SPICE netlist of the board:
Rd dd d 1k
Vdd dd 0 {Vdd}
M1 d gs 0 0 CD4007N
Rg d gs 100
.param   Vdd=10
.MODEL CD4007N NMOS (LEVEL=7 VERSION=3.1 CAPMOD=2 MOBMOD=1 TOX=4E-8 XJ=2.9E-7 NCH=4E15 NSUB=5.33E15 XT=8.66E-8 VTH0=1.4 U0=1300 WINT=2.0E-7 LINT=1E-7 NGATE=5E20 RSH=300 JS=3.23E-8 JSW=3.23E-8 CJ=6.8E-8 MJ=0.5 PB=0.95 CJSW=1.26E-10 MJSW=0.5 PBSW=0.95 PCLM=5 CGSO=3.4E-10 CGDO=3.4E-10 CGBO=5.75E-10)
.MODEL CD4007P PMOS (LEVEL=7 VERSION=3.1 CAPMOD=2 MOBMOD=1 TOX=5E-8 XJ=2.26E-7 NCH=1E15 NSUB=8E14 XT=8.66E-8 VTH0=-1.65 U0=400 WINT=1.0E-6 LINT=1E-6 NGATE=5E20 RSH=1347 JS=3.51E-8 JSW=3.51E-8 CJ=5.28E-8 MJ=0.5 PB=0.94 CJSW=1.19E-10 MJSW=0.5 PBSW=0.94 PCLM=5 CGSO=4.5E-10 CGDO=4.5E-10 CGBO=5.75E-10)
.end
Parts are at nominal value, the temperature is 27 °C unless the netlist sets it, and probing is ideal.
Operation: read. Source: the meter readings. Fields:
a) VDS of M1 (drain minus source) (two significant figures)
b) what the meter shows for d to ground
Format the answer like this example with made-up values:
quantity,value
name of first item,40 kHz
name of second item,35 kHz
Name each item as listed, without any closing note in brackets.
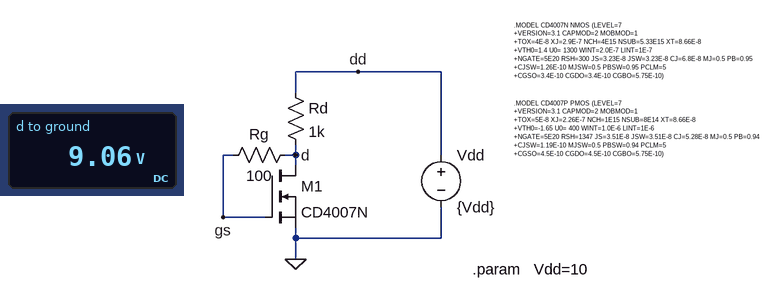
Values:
quantity,value
VDS of M1 (drain minus source),9.1 V
what the meter shows for d to ground,9.06 V
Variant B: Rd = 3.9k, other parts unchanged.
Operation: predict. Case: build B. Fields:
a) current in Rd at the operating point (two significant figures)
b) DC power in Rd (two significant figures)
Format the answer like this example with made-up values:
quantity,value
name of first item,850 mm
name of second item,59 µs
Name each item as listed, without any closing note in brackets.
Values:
quantity,value
current in Rd at the operating point,650 µA
DC power in Rd,1.7 mW
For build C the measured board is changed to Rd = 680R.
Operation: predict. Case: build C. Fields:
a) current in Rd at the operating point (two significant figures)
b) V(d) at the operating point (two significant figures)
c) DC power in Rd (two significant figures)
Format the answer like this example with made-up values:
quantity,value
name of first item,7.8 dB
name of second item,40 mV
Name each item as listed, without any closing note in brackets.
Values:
quantity,value
current in Rd at the operating point,990 µA
V(d) at the operating point,9.3 V
DC power in Rd,660 µW
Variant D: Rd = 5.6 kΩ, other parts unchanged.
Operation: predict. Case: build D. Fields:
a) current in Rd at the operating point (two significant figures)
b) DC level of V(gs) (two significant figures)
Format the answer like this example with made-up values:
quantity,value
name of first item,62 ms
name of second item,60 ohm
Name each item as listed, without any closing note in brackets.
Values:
quantity,value
current in Rd at the operating point,560 µA
DC level of V(gs),6.9 V
